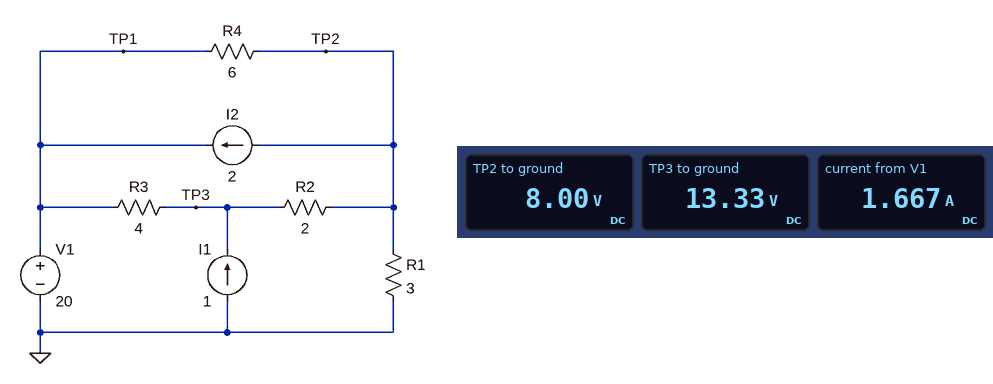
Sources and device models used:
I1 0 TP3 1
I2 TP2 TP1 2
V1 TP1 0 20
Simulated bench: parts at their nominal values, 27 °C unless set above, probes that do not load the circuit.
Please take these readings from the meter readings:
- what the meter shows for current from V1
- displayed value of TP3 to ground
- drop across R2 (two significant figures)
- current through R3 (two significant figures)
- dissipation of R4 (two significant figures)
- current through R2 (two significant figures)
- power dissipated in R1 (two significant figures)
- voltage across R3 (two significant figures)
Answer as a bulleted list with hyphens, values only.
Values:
- 1.667 A
- 13.33 V
- 5.3 V
- 1.7 A
- 24 W
- 2.7 A
- 21 W
- 6.7 V
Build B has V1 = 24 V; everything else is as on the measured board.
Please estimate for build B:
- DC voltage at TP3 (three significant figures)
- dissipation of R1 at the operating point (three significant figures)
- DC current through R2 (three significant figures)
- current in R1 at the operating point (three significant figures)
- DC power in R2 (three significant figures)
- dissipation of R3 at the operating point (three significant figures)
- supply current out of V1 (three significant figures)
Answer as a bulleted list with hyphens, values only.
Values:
- 16.0 V
- 33.3 W
- 3.00 A
- 3.33 A
- 18.0 W
- 16.0 W
- 2.33 A
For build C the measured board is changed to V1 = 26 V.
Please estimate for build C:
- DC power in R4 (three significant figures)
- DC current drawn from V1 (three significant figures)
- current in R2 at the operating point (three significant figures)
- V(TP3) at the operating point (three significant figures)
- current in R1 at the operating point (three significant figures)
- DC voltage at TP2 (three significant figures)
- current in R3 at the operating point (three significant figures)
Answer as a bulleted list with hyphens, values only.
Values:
- 37.5 W
- 2.67 A
- 3.17 A
- 17.3 V
- 3.67 A
- 11.0 V
- 2.17 A
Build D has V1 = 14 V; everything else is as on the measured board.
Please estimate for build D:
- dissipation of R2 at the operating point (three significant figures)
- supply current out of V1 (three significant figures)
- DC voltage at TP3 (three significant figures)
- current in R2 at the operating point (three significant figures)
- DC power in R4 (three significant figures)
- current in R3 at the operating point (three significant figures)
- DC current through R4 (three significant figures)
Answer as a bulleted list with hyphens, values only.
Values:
- 9.39 W
- 667 mA
- 9.33 V
- 2.17 A
- 13.5 W
- 1.17 A
- 1.50 A
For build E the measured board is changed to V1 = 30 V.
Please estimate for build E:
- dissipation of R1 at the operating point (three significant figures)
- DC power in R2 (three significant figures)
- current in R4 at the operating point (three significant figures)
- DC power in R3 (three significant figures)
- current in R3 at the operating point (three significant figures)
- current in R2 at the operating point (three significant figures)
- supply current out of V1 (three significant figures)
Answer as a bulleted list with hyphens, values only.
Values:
- 56.3 W
- 24.5 W
- 2.83 A
- 25.0 W
- 2.50 A
- 3.50 A
- 3.33 A
